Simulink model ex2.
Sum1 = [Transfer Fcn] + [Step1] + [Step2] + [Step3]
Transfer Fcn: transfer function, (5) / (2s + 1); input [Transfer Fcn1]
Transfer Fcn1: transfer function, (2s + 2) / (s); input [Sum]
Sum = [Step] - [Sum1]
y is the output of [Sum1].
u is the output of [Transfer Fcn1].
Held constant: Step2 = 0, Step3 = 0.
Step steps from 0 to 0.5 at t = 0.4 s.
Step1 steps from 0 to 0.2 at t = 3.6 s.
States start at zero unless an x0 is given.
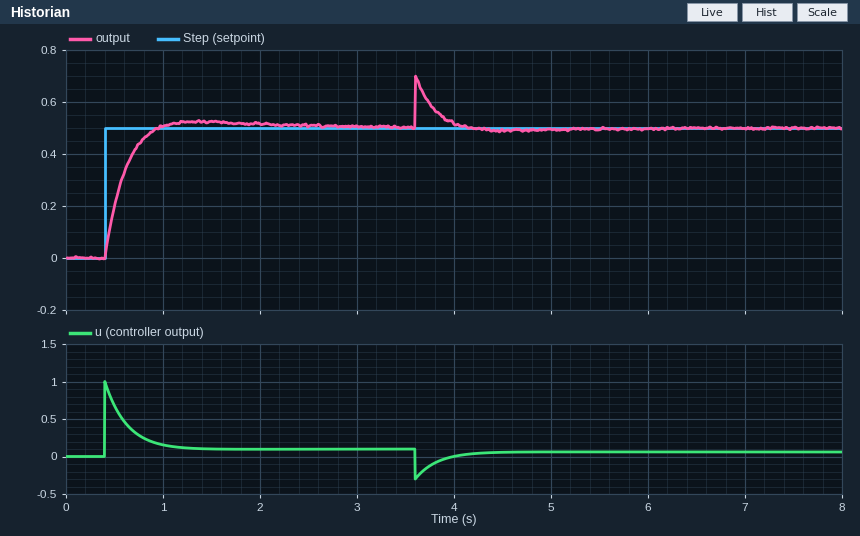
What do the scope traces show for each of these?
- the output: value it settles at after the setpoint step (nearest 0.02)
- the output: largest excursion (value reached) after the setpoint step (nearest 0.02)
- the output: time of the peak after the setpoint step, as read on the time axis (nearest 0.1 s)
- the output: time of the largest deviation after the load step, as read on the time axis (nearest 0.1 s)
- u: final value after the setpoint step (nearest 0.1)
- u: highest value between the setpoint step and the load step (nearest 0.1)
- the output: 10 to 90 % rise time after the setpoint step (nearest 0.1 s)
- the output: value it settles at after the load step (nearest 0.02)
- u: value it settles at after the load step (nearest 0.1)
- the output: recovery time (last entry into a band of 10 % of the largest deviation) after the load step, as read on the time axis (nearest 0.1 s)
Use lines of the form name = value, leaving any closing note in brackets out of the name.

the output: value it settles at after the setpoint step = 0.50
the output: largest excursion (value reached) after the setpoint step = 0.52
the output: time of the peak after the setpoint step, as read on the time axis = 1.4 s
the output: time of the largest deviation after the load step, as read on the time axis = 3.6 s
u: final value after the setpoint step = 0.1
u: highest value between the setpoint step and the load step = 1.0
the output: 10 to 90 % rise time after the setpoint step = 0.4 s
the output: value it settles at after the load step = 0.50
u: value it settles at after the load step = 0.1
the output: recovery time (last entry into a band of 10 % of the largest deviation) after the load step, as read on the time axis = 4.0 s
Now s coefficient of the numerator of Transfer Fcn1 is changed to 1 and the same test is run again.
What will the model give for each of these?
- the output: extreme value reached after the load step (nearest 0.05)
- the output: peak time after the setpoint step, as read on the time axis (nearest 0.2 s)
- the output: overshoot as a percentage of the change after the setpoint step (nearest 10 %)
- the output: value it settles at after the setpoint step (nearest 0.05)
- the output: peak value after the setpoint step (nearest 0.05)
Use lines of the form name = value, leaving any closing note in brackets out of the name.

the output: extreme value reached after the load step = 0.70
the output: peak time after the setpoint step, as read on the time axis = 1.6 s
the output: overshoot as a percentage of the change after the setpoint step = 20 %
the output: value it settles at after the setpoint step = 0.50
the output: peak value after the setpoint step = 0.60
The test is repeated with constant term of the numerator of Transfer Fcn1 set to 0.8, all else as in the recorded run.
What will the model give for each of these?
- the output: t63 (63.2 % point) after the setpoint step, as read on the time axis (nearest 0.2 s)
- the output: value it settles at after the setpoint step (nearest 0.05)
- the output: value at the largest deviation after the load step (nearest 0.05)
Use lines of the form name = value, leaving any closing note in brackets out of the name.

the output: t63 (63.2 % point) after the setpoint step, as read on the time axis = 0.6 s
the output: value it settles at after the setpoint step = 0.50
the output: value at the largest deviation after the load step = 0.70
